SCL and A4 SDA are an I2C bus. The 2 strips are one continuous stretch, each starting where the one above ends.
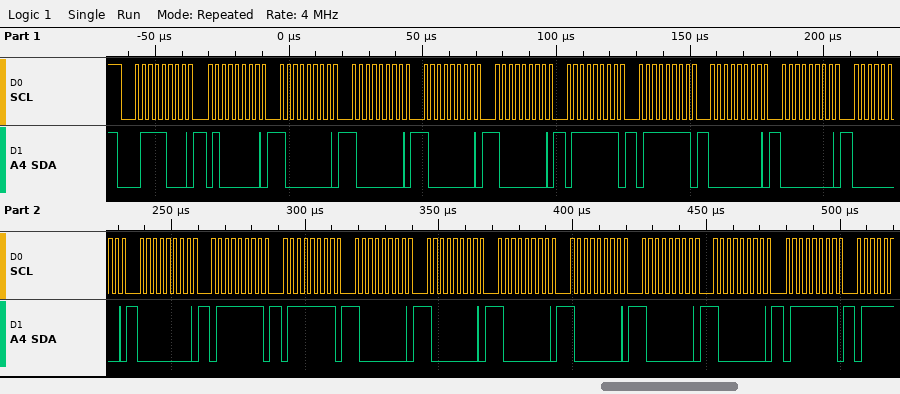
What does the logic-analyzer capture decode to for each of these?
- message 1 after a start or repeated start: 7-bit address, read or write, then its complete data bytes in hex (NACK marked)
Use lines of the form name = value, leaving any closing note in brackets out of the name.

message 1 after a start or repeated start: 7-bit address, read or write, then its complete data bytes in hex = 0x3C write: 40 80 80 80 80 7F 7F 00 00 00 00 7F 7F 80 80 80 80 80 80 7F
